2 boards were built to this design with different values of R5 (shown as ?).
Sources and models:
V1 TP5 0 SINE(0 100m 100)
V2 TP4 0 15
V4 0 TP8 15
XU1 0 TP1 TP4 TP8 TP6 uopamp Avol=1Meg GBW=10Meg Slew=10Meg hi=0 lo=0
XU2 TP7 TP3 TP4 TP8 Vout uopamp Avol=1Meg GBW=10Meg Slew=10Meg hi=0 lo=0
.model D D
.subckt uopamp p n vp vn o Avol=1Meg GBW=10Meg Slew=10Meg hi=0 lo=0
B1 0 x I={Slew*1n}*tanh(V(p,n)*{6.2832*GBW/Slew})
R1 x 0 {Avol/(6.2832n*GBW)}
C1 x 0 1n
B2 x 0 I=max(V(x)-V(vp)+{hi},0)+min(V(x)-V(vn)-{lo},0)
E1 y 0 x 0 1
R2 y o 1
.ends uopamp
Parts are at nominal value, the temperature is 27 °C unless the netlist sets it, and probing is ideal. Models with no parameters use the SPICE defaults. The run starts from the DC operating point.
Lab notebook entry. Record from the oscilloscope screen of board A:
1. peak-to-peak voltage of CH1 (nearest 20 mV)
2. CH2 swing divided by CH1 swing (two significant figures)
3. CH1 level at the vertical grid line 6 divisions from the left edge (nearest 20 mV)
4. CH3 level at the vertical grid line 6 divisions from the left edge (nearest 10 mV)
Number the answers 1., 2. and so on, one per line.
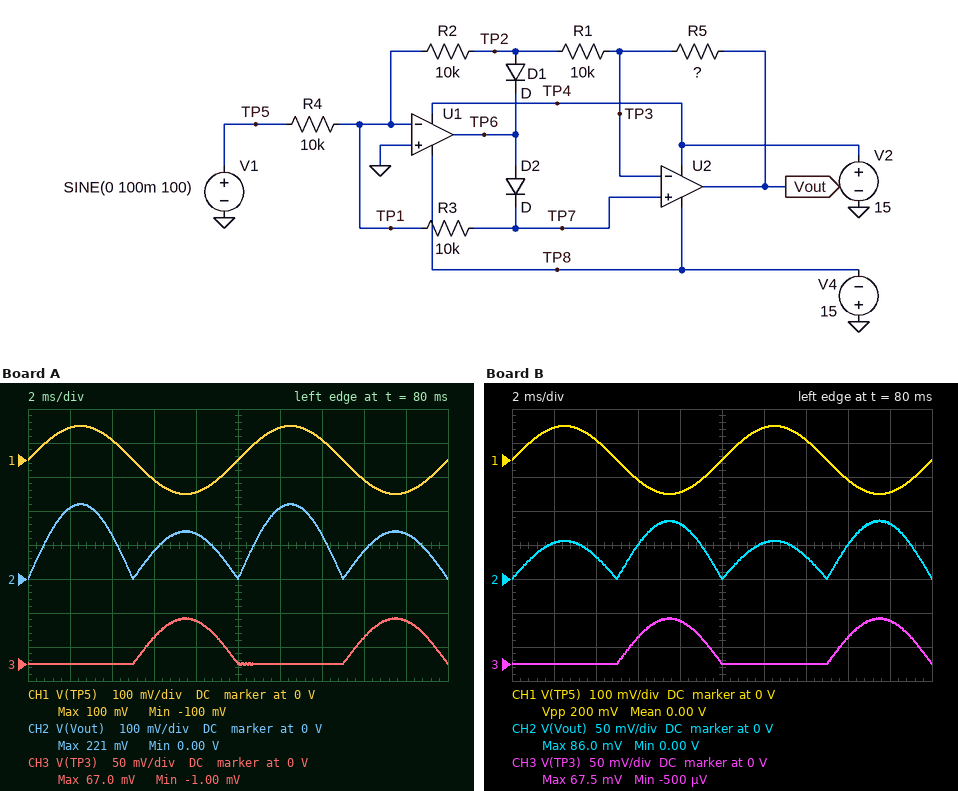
1. 200 mV
2. 1.1
3. 100 mV
4. 0 V
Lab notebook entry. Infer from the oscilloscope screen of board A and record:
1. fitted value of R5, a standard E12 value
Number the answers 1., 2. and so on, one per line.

1. 22 kΩ
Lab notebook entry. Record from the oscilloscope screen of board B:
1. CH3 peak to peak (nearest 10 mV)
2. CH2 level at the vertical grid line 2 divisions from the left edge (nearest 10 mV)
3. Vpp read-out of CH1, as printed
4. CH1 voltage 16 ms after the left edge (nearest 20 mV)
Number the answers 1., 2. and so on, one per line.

1. 70 mV
2. 30 mV
3. 200 mV
4. -60 mV
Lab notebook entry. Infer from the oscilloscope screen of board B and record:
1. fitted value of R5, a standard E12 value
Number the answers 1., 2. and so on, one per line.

1. 5.6 kΩ
